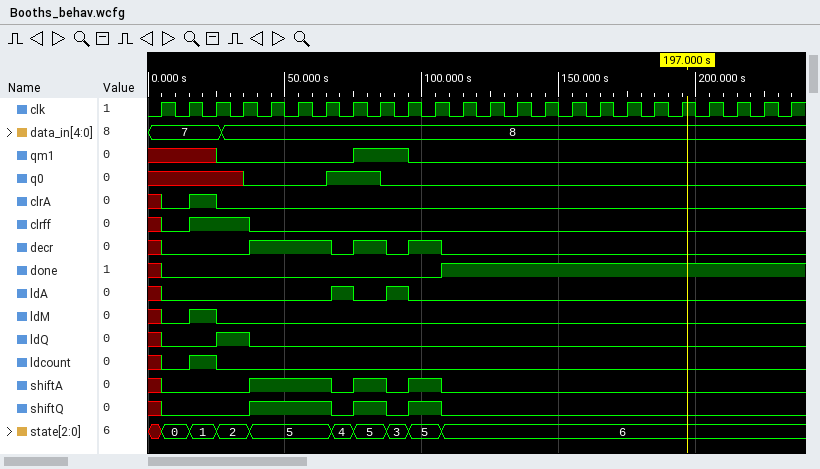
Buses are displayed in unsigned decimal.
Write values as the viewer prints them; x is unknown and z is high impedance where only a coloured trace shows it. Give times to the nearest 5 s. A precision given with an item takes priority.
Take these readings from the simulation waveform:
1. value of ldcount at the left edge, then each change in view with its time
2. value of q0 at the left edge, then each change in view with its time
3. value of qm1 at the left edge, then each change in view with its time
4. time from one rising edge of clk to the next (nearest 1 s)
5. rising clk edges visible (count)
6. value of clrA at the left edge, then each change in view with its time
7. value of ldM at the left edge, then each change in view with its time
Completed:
x, 0 at 5 s, 1 at 15 s, 0 at 25 s
x, 0 at 35 s, 1 at 65 s, 0 at 85 s
x, 0 at 25 s, 1 at 75 s, 0 at 95 s
10 s
24
x, 0 at 5 s, 1 at 15 s, 0 at 25 s
x, 0 at 5 s, 1 at 15 s, 0 at 25 s
